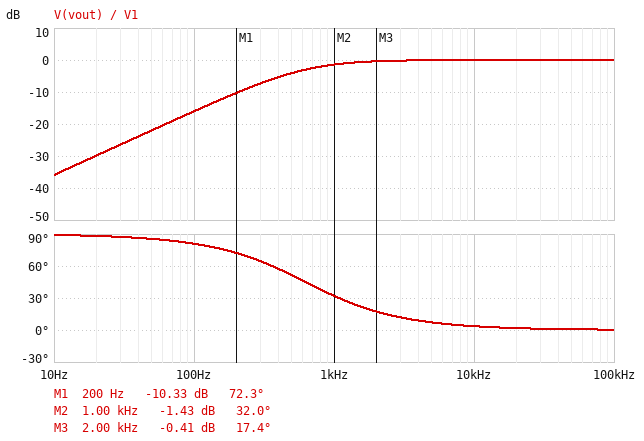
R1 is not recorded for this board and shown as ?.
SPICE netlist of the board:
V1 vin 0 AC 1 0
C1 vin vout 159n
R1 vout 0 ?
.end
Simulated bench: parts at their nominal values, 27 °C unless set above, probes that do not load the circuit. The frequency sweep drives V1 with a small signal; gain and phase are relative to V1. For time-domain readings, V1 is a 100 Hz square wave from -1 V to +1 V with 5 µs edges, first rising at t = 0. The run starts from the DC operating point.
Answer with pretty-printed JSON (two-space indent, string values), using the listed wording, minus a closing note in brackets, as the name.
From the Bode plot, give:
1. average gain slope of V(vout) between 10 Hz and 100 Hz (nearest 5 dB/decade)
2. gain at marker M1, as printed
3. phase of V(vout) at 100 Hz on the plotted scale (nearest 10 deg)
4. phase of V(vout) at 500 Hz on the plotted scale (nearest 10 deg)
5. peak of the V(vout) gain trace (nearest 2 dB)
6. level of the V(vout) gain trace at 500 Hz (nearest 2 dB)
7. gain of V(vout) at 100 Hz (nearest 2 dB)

{
  "average gain slope of V(vout) between 10 Hz and 100 Hz": "20 dB/decade",
  "gain at marker M1, as printed": "-10.33 dB",
  "phase of V(vout) at 100 Hz on the plotted scale": "80 deg",
  "phase of V(vout) at 500 Hz on the plotted scale": "50 deg",
  "peak of the V(vout) gain trace": "0 dB",
  "level of the V(vout) gain trace at 500 Hz": "-4 dB",
  "gain of V(vout) at 100 Hz": "-16 dB"
}
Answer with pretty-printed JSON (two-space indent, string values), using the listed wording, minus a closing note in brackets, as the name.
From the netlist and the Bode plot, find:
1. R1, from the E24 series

{
  "R1, from the E24 series": "1.6 kΩ"
}
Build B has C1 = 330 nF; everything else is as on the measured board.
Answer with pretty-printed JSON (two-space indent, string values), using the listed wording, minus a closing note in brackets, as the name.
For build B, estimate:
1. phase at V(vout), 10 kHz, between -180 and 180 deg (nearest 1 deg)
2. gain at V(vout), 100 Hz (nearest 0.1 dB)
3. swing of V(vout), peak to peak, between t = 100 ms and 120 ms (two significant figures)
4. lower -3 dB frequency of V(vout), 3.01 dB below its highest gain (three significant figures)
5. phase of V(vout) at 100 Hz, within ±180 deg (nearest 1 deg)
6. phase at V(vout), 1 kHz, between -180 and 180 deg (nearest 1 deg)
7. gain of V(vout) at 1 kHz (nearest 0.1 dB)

{
  "phase at V(vout), 10 kHz, between -180 and 180 deg": "2 deg",
  "gain at V(vout), 100 Hz": "-10.0 dB",
  "swing of V(vout), peak to peak, between t = 100 ms and 120 ms": "4.0 V",
  "lower -3 dB frequency of V(vout), 3.01 dB below its highest gain": "301 Hz",
  "phase of V(vout) at 100 Hz, within ±180 deg": "72 deg",
  "phase at V(vout), 1 kHz, between -180 and 180 deg": "17 deg",
  "gain of V(vout) at 1 kHz": "-0.4 dB"
}
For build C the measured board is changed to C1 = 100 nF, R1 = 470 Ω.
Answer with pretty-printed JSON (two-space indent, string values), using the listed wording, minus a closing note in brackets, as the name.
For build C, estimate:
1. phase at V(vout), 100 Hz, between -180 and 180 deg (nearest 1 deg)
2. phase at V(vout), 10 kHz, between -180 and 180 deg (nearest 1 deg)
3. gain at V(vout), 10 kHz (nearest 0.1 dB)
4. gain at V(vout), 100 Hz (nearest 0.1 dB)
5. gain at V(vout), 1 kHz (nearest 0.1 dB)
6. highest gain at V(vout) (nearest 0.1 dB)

{
  "phase at V(vout), 100 Hz, between -180 and 180 deg": "88 deg",
  "phase at V(vout), 10 kHz, between -180 and 180 deg": "19 deg",
  "gain at V(vout), 10 kHz": "-0.5 dB",
  "gain at V(vout), 100 Hz": "-30.6 dB",
  "gain at V(vout), 1 kHz": "-11.0 dB",
  "highest gain at V(vout)": "0 dB"
}
